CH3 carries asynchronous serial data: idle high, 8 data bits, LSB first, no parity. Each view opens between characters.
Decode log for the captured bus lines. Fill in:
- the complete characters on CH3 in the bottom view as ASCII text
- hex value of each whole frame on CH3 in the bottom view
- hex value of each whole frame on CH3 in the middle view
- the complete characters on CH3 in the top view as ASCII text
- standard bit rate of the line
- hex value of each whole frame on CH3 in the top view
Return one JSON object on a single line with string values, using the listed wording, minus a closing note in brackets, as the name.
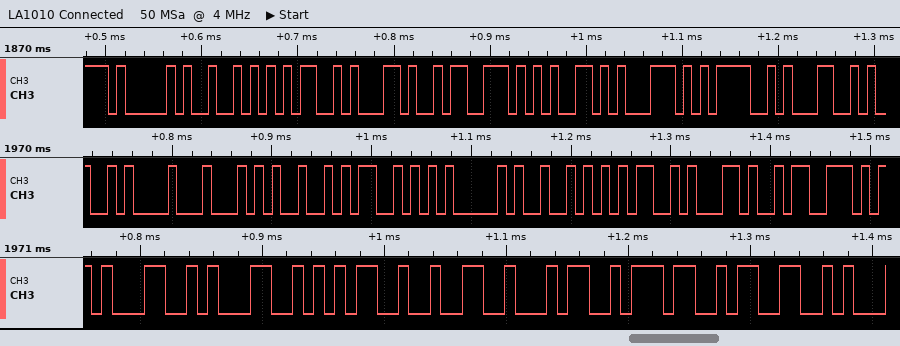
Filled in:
{"the complete characters on CH3 in the bottom view as ASCII text": "\"1152473\"", "hex value of each whole frame on CH3 in the bottom view": "31, 31, 35, 32, 34, 37, 33", "hex value of each whole frame on CH3 in the middle view": "0A, 44, 49, 53, 41, 52, 4D, 2C, 73", "the complete characters on CH3 in the top view as ASCII text": "\"ARM,seq=1\"", "standard bit rate of the line": "115200 baud", "hex value of each whole frame on CH3 in the top view": "41, 52, 4D, 2C, 73, 65, 71, 3D, 31"}
